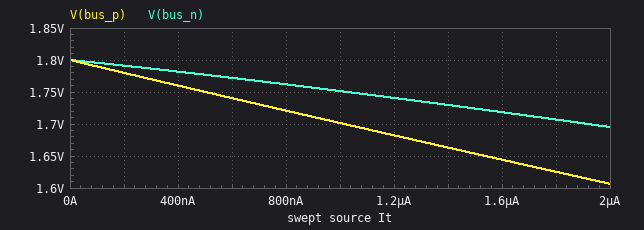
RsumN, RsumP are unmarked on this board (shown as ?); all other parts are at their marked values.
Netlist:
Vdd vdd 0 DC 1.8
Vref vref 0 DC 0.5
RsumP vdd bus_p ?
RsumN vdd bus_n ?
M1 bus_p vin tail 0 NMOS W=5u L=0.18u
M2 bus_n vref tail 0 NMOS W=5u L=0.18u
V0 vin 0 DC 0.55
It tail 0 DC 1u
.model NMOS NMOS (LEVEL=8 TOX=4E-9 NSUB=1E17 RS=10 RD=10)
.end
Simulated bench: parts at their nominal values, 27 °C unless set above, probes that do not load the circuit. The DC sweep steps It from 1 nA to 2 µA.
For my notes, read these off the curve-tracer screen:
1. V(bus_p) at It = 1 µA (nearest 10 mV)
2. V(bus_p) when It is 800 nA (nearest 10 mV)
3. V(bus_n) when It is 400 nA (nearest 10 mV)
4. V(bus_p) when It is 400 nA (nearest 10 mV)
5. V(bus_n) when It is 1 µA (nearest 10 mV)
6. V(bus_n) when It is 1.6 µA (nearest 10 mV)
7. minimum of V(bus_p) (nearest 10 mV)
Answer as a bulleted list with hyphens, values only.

- 1.70 V
- 1.72 V
- 1.78 V
- 1.76 V
- 1.75 V
- 1.72 V
- 1.61 V
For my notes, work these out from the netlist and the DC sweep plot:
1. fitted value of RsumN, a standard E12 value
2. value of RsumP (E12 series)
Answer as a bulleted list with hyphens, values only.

- 270 kΩ
- 120 kΩ
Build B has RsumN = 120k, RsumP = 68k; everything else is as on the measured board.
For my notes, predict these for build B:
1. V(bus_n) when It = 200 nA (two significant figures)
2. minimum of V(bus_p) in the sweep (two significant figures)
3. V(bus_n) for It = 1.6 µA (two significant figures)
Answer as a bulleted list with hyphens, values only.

- 1.8 V
- 1.7 V
- 1.8 V
